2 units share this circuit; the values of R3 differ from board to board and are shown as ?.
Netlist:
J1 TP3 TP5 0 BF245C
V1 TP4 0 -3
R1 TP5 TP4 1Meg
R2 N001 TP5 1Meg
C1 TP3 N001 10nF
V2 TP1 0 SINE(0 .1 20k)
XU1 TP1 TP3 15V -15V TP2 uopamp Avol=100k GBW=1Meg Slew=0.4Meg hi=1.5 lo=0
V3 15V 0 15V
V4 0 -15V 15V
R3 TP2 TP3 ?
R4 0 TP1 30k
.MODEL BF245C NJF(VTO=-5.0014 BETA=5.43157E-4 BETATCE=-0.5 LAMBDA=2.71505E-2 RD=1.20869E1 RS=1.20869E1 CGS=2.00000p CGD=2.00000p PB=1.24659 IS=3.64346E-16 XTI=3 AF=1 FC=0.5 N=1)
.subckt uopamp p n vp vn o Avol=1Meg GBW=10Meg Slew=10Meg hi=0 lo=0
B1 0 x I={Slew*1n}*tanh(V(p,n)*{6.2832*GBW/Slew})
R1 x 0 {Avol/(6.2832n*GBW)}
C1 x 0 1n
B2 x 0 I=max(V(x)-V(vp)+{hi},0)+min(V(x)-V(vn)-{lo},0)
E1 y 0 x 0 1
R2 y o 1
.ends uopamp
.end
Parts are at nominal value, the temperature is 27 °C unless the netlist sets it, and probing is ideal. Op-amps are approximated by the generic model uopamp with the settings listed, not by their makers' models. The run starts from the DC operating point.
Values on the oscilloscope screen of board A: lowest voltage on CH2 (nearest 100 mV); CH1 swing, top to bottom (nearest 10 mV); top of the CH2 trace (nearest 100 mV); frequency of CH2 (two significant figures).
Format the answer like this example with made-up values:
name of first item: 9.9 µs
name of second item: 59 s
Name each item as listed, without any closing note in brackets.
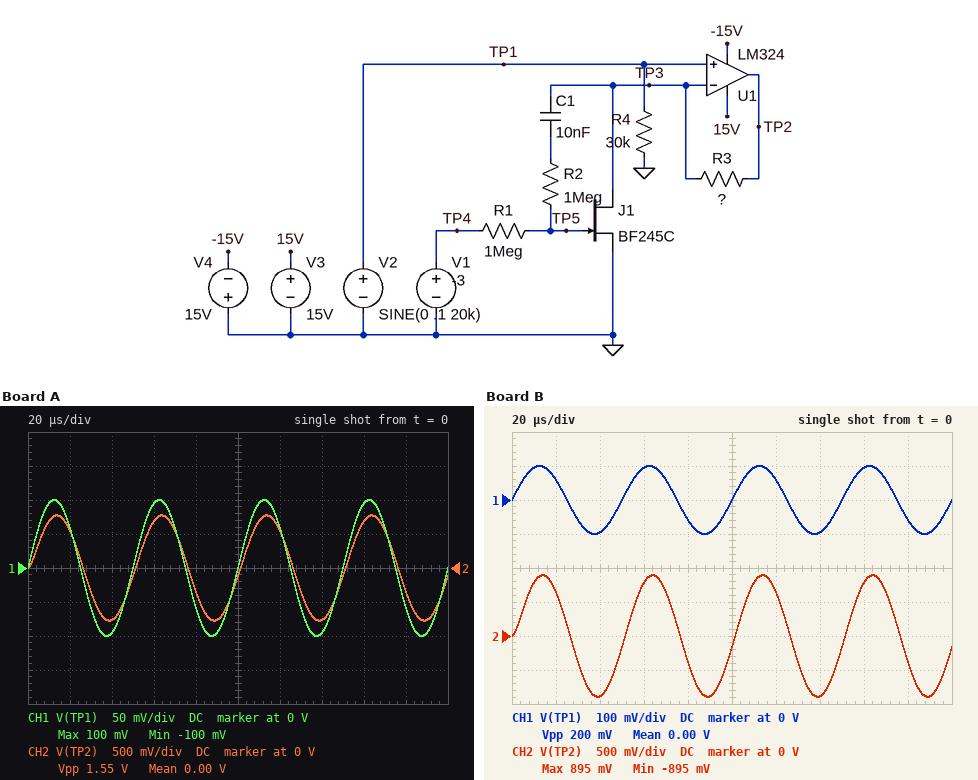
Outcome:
lowest voltage on CH2: -800 mV
CH1 swing, top to bottom: 200 mV
top of the CH2 trace: 800 mV
frequency of CH2: 20 kHz
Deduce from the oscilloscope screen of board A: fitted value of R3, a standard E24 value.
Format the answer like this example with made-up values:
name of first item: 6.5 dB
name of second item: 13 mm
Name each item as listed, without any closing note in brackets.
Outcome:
fitted value of R3, a standard E24 value: 3.3 kΩ
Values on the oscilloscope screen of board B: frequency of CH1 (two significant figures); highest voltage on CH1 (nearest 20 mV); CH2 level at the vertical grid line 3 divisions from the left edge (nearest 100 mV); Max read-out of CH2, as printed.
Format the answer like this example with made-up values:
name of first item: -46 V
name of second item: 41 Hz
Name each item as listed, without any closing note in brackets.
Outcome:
frequency of CH1: 20 kHz
highest voltage on CH1: 100 mV
CH2 level at the vertical grid line 3 divisions from the left edge: 800 mV
Max read-out of CH2, as printed: 895 mV
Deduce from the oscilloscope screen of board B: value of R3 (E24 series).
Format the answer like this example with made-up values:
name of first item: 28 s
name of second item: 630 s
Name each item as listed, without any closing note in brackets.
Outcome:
value of R3: 3.9 kΩ
